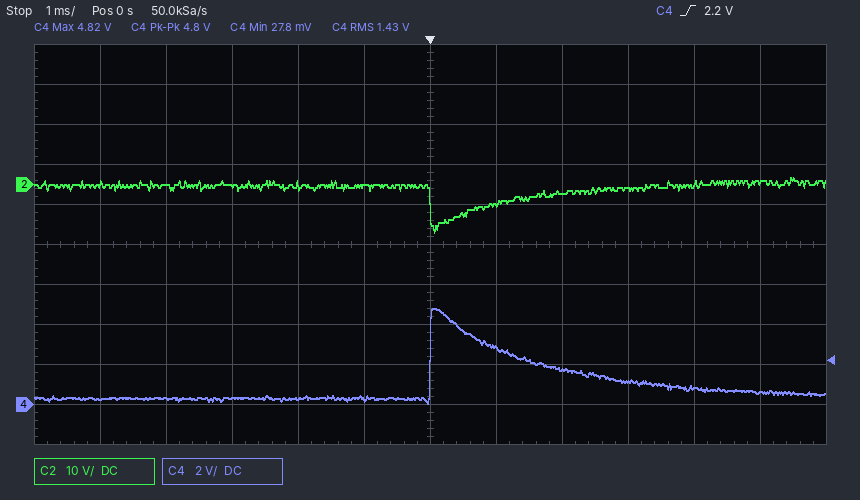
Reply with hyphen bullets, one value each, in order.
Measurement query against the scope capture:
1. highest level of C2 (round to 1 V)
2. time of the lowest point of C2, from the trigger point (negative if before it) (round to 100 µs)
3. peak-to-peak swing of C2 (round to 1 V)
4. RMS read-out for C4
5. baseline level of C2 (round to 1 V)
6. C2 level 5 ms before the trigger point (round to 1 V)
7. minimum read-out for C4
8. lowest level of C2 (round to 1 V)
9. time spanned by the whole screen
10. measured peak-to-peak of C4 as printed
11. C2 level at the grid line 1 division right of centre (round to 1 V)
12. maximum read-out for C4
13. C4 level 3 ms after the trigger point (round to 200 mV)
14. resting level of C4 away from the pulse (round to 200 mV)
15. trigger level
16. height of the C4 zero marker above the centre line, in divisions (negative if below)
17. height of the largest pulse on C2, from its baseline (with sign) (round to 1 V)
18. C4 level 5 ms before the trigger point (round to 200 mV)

- 2 V
- +100 µs
- 14 V
- 1.43 V
- 0 V
- 0 V
- 27.8 mV
- -12 V
- 12 ms
- 4.8 V
- -5 V
- 4.82 V
- 1.2 V
- 400 mV
- 2.2 V
- -4.0 div
- -12 V
- 200 mV
